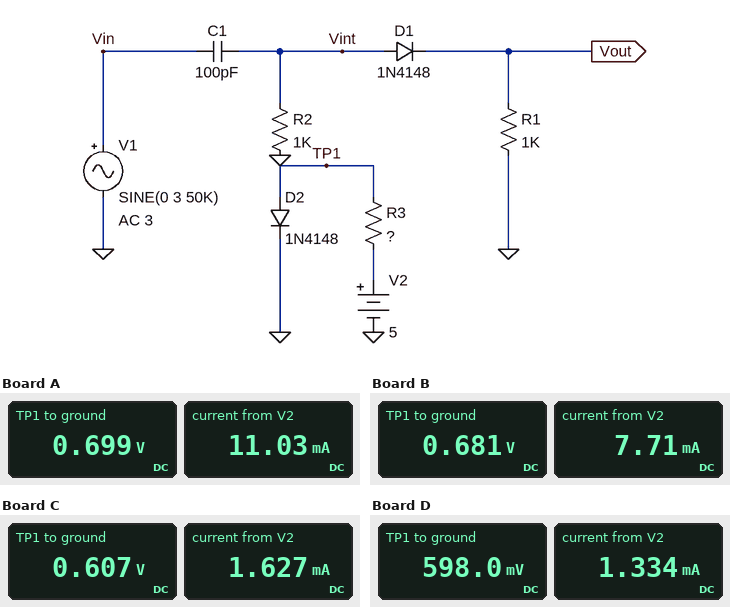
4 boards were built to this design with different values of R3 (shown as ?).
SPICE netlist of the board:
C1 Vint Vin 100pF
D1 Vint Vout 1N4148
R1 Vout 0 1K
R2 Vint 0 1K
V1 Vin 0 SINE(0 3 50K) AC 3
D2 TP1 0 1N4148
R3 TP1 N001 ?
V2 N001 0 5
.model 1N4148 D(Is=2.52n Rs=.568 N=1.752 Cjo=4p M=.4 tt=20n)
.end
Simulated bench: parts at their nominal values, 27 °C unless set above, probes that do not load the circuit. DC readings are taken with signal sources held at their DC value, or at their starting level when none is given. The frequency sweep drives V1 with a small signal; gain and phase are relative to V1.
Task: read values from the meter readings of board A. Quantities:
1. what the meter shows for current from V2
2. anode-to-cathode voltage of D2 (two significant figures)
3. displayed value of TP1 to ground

11.03 mA
700 mV
0.699 V
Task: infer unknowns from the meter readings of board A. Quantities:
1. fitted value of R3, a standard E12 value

390 Ω
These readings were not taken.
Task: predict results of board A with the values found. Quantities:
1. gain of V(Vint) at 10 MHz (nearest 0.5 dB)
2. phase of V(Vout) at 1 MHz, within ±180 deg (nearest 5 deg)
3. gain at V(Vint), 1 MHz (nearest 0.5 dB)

-0.5 dB
145 deg
-5.5 dB
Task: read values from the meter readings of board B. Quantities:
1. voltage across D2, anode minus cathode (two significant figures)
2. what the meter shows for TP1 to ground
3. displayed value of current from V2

680 mV
0.681 V
7.71 mA
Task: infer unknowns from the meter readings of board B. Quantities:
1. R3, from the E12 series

560 Ω
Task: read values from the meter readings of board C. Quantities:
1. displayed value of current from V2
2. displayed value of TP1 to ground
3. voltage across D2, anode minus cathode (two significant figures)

1.627 mA
0.607 V
610 mV
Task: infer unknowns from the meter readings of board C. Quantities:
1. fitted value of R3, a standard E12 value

2.7 kΩ
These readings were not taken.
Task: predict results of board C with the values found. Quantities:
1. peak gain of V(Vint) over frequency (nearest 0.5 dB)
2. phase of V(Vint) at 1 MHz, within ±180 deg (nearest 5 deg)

0 dB
55 deg
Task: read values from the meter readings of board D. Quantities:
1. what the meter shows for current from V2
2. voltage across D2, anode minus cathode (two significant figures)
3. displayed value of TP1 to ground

1.334 mA
600 mV
598.0 mV
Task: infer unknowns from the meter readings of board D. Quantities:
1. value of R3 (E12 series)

3.3 kΩ
